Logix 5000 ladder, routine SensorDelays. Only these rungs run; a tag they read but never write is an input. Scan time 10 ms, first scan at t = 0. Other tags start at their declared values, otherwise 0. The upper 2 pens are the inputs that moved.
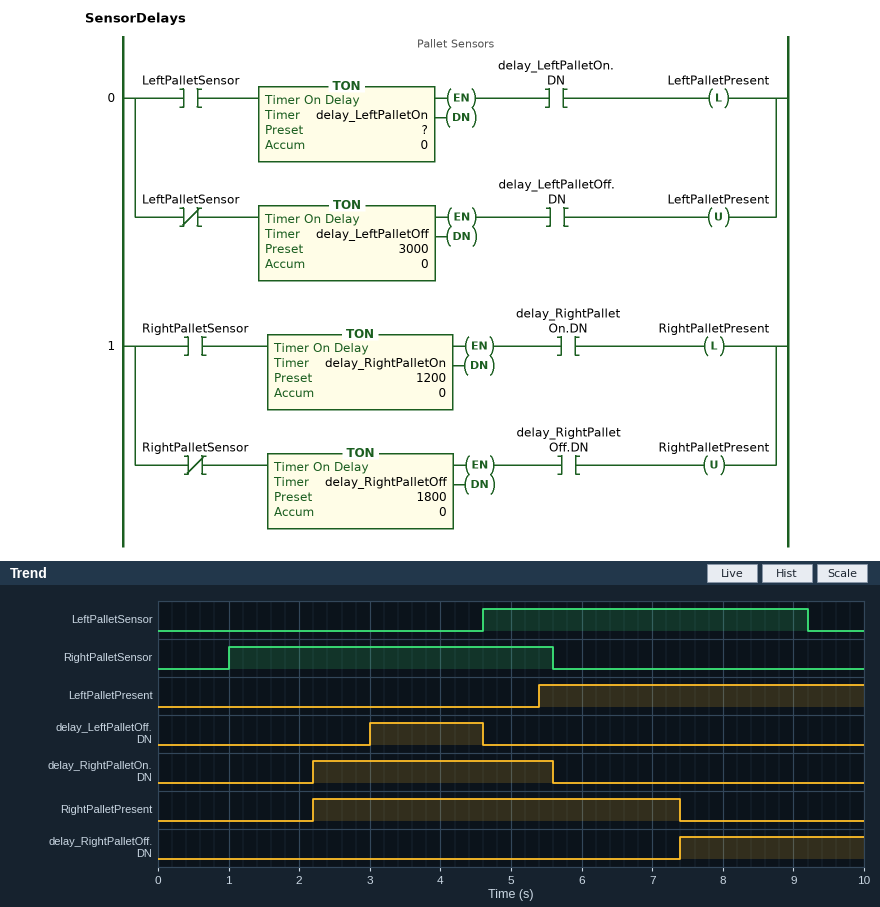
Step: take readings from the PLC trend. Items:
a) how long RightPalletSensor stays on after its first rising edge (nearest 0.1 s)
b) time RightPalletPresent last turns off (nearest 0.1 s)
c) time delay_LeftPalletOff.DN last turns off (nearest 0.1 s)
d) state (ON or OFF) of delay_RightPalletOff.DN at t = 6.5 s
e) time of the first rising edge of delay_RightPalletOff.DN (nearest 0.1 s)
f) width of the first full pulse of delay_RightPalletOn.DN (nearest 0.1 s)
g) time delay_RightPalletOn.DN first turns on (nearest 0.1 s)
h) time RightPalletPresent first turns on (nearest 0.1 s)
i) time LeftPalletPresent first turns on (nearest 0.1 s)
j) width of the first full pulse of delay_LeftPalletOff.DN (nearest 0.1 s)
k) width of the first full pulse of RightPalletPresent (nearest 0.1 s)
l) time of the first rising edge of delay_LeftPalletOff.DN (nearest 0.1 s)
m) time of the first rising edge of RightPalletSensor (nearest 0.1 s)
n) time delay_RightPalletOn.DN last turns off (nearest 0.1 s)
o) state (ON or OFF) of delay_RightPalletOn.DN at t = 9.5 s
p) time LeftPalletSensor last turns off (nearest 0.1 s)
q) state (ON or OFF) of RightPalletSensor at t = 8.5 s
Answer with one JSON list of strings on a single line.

["4.6 s", "7.4 s", "4.6 s", "OFF", "7.4 s", "3.4 s", "2.2 s", "2.2 s", "5.4 s", "1.6 s", "5.2 s", "3.0 s", "1.0 s", "5.6 s", "OFF", "9.2 s", "OFF"]
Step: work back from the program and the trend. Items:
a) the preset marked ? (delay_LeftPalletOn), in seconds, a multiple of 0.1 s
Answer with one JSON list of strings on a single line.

["0.8 s"]
